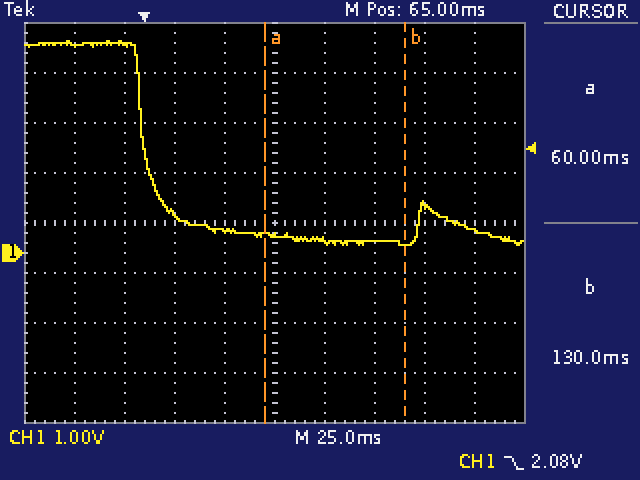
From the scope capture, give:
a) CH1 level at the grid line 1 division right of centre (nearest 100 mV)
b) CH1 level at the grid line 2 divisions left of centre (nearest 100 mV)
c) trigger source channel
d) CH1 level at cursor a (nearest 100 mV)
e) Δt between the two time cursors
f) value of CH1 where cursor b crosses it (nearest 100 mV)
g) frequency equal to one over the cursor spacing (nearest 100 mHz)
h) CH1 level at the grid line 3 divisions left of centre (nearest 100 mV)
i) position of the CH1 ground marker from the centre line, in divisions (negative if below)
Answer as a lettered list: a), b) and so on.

a) 200 mV
b) 800 mV
c) CH1
d) 400 mV
e) 70.0 ms
f) 200 mV
g) 14.3 Hz
h) 4.2 V
i) -0.6 div
